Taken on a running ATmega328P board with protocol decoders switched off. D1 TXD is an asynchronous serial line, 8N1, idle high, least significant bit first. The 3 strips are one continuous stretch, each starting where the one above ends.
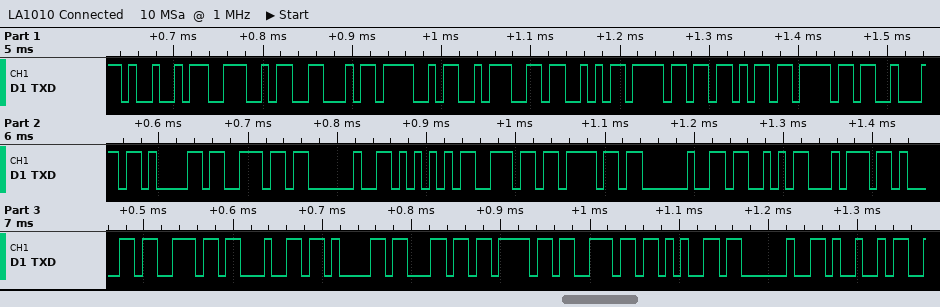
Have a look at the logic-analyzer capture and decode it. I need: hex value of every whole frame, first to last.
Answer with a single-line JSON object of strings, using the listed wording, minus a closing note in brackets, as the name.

{"hex value of every whole frame, first to last": "49 4E 46 4F 3A 53 6F 6B 6F 62 61 6E 20 55 6E 6F 20 53 74 61 6E 64 61 6C 6F 6E 65 20 49"}
